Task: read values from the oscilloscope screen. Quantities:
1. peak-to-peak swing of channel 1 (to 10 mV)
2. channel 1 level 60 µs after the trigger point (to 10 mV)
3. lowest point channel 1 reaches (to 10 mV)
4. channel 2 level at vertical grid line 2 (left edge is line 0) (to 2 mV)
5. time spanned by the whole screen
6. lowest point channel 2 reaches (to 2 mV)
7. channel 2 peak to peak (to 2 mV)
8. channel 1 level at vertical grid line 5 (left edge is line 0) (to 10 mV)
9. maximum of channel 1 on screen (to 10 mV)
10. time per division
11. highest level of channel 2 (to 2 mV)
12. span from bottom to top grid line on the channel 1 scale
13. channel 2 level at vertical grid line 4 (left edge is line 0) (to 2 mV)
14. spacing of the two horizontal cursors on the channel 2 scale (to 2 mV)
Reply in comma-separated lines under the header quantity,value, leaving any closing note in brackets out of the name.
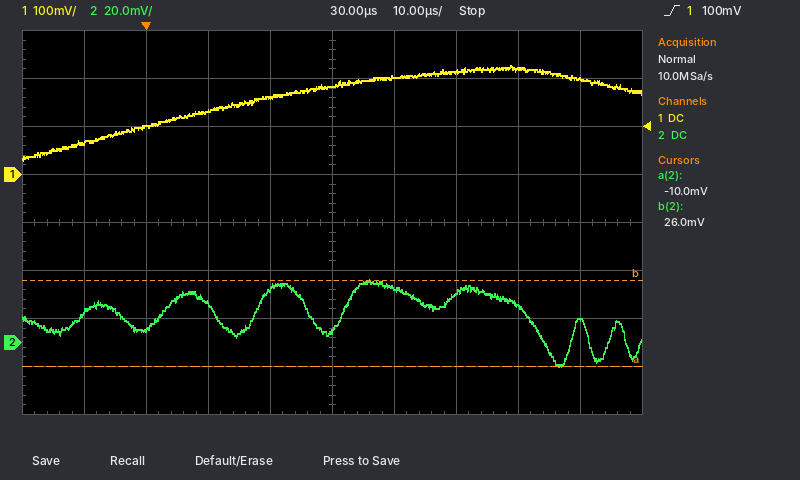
quantity,value
peak-to-peak swing of channel 1,200 mV
channel 1 level 60 µs after the trigger point,220 mV
lowest point channel 1 reaches,30 mV
channel 2 level at vertical grid line 2 (left edge is line 0),6 mV
time spanned by the whole screen,100 µs
lowest point channel 2 reaches,-10 mV
channel 2 peak to peak,36 mV
channel 1 level at vertical grid line 5 (left edge is line 0),180 mV
maximum of channel 1 on screen,230 mV
time per division,10 µs
highest level of channel 2,26 mV
span from bottom to top grid line on the channel 1 scale,800 mV
channel 2 level at vertical grid line 4 (left edge is line 0),22 mV
spacing of the two horizontal cursors on the channel 2 scale,36 mV
